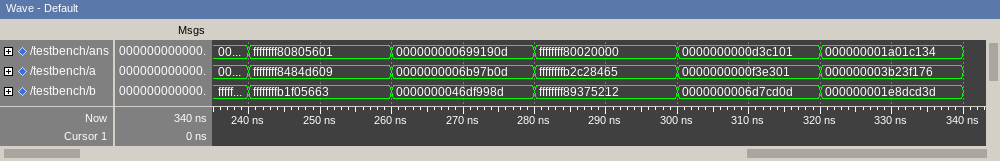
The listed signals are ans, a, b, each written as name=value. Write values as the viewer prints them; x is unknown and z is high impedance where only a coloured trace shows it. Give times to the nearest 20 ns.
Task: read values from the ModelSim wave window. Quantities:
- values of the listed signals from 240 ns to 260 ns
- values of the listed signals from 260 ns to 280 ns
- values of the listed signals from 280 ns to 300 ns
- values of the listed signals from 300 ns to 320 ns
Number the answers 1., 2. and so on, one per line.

1. ans=ffffffff80805601, a=ffffffff8484d609, b=ffffffffb1f05663
2. ans=000000000699190d, a=0000000006b97b0d, b=0000000046df998d
3. ans=ffffffff80020000, a=ffffffffb2c28465, b=ffffffff89375212
4. ans=0000000000d3c101, a=0000000000f3e301, b=0000000006d7cd0d
